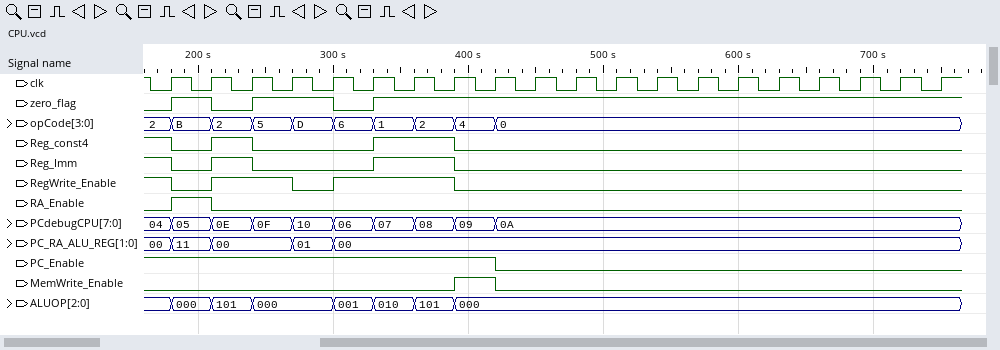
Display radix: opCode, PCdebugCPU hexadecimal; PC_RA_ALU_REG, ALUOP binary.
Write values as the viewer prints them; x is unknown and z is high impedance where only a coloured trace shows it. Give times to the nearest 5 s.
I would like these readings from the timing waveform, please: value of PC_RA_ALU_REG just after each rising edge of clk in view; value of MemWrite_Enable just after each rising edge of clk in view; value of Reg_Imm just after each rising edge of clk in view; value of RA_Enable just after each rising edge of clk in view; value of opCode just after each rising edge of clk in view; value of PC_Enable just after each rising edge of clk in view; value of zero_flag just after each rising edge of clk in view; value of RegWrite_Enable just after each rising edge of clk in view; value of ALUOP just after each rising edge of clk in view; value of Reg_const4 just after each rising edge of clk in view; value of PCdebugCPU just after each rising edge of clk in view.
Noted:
11, 00, 00, 01, 00, 00, 00, 00, 00, 00, 00, 00, 00, 00, 00, 00, 00, 00, 00, 00
0 0 0 0 0 0 0 1 0 0 0 0 0 0 0 0 0 0 0 0
0 1 0 0 0 1 1 0 0 0 0 0 0 0 0 0 0 0 0 0
1 0 0 0 0 0 0 0 0 0 0 0 0 0 0 0 0 0 0 0
B, 2, 5, D, 6, 1, 2, 4, 0, 0, 0, 0, 0, 0, 0, 0, 0, 0, 0, 0
1 1 1 1 1 1 1 1 0 0 0 0 0 0 0 0 0 0 0 0
1 0 1 1 0 1 1 1 1 1 1 1 1 1 1 1 1 1 1 1
0 1 1 0 1 1 1 0 0 0 0 0 0 0 0 0 0 0 0 0
000, 101, 000, 000, 001, 010, 101, 000, 000, 000, 000, 000, 000, 000, 000, 000, 000, 000, 000, 000
0 1 0 0 0 1 1 0 0 0 0 0 0 0 0 0 0 0 0 0
05, 0E, 0F, 10, 06, 07, 08, 09, 0A, 0A, 0A, 0A, 0A, 0A, 0A, 0A, 0A, 0A, 0A, 0A
